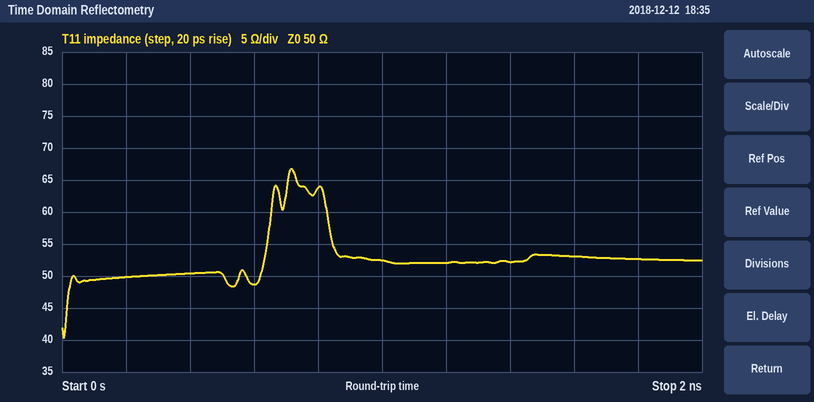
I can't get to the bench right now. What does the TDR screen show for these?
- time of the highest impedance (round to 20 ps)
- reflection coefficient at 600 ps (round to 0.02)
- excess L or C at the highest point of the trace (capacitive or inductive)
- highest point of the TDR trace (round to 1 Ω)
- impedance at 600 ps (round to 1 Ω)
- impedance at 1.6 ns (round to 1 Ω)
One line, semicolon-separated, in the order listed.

720 ps; -0.02; inductive; 67 Ω; 49 Ω; 53 Ω
